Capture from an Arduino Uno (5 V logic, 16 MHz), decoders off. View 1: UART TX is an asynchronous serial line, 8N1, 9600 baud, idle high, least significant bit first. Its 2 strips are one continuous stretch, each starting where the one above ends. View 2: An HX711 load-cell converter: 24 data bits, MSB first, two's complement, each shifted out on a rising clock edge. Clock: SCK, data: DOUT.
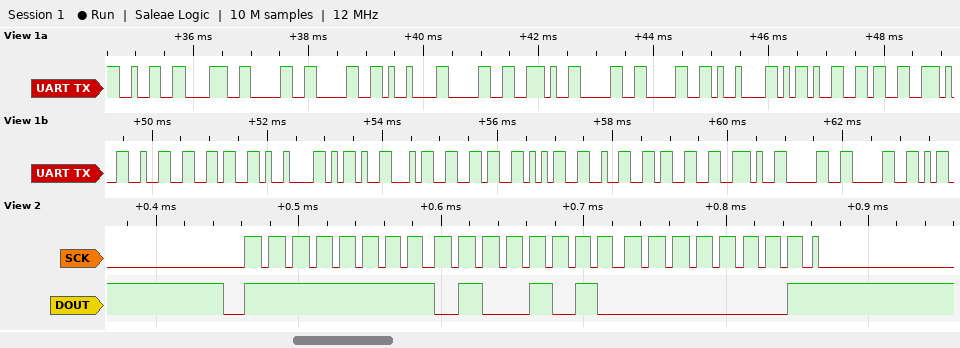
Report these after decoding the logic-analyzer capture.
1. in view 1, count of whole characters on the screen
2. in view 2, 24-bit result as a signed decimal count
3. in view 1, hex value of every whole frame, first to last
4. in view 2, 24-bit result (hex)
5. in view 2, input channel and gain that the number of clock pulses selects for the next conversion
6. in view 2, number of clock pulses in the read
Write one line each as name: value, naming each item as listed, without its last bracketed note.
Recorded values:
in view 1, count of whole characters on the screen: 25
in view 2, 24-bit result as a signed decimal count: -46591
in view 1, hex value of every whole frame, first to last: 32 38 30 30 09 30 2E 30 30 09 2D 36 2E 32 36 09 2D 34 36 35 32 33 2E 30 30
in view 2, 24-bit result: 0xFF4A01
in view 2, input channel and gain that the number of clock pulses selects for the next conversion: channel A, gain 128
in view 2, number of clock pulses in the read: 25
